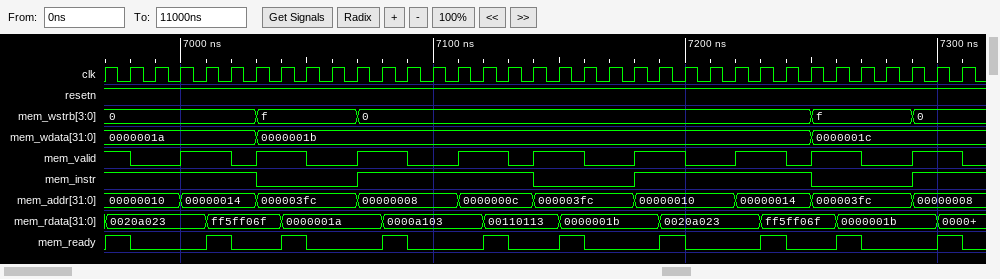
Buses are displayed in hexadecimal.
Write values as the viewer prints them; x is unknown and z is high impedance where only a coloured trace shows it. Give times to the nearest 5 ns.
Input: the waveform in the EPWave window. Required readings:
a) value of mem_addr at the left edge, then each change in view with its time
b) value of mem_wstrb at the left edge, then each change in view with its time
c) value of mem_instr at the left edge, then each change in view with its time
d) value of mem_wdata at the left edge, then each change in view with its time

00000010, 00000014 at 7000 ns, 000003fc at 7030 ns, 00000008 at 7070 ns, 0000000c at 7110 ns, 000003fc at 7140 ns, 00000010 at 7180 ns, 00000014 at 7220 ns, 000003fc at 7250 ns, 00000008 at 7290 ns
0, f at 7030 ns, 0 at 7070 ns, f at 7250 ns, 0 at 7290 ns
1, 0 at 7030 ns, 1 at 7070 ns, 0 at 7140 ns, 1 at 7180 ns, 0 at 7250 ns, 1 at 7290 ns
0000001a, 0000001b at 7030 ns, 0000001c at 7250 ns
